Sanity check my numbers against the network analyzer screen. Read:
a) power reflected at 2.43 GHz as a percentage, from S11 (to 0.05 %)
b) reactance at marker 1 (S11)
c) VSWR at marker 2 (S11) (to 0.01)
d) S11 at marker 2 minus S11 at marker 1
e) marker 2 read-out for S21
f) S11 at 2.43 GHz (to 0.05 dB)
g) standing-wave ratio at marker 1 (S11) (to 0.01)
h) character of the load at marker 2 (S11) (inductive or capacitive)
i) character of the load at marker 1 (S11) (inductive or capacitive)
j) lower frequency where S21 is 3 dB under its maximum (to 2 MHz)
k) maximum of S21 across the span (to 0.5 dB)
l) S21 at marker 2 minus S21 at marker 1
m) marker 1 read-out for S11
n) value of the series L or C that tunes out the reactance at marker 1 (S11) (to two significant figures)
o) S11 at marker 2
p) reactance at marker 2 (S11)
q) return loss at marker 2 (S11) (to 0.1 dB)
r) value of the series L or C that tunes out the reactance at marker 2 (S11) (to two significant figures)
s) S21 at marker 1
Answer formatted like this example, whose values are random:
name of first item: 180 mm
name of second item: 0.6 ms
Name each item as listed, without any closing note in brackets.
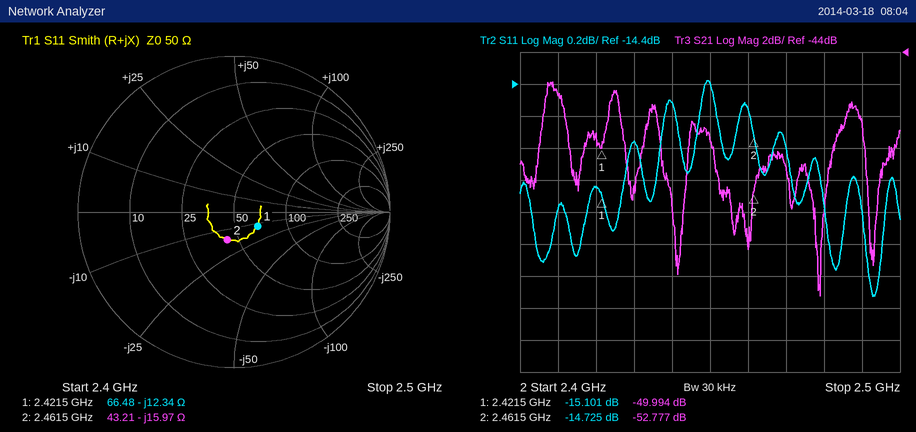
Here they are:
power reflected at 2.43 GHz as a percentage, from S11: 3.35 %
reactance at marker 1: -12.34 Ω
VSWR at marker 2 (S11): 1.45
S11 at marker 2 minus S11 at marker 1: 0.376 dB
marker 2 read-out for S21: -52.777 dB
S11 at 2.43 GHz: -14.75 dB
standing-wave ratio at marker 1 (S11): 1.43
character of the load at marker 2 (S11): capacitive
character of the load at marker 1 (S11): capacitive
lower frequency where S21 is 3 dB under its maximum: 2.406 GHz
maximum of S21 across the span: -46.0 dB
S21 at marker 2 minus S21 at marker 1: -2.783 dB
marker 1 read-out for S11: -15.101 dB
value of the series L or C that tunes out the reactance at marker 1 (S11): 810 pH
S11 at marker 2: -14.725 dB
reactance at marker 2: -15.97 Ω
return loss at marker 2 (S11): 14.7 dB
value of the series L or C that tunes out the reactance at marker 2 (S11): 1.0 nH
S21 at marker 1: -49.994 dB
